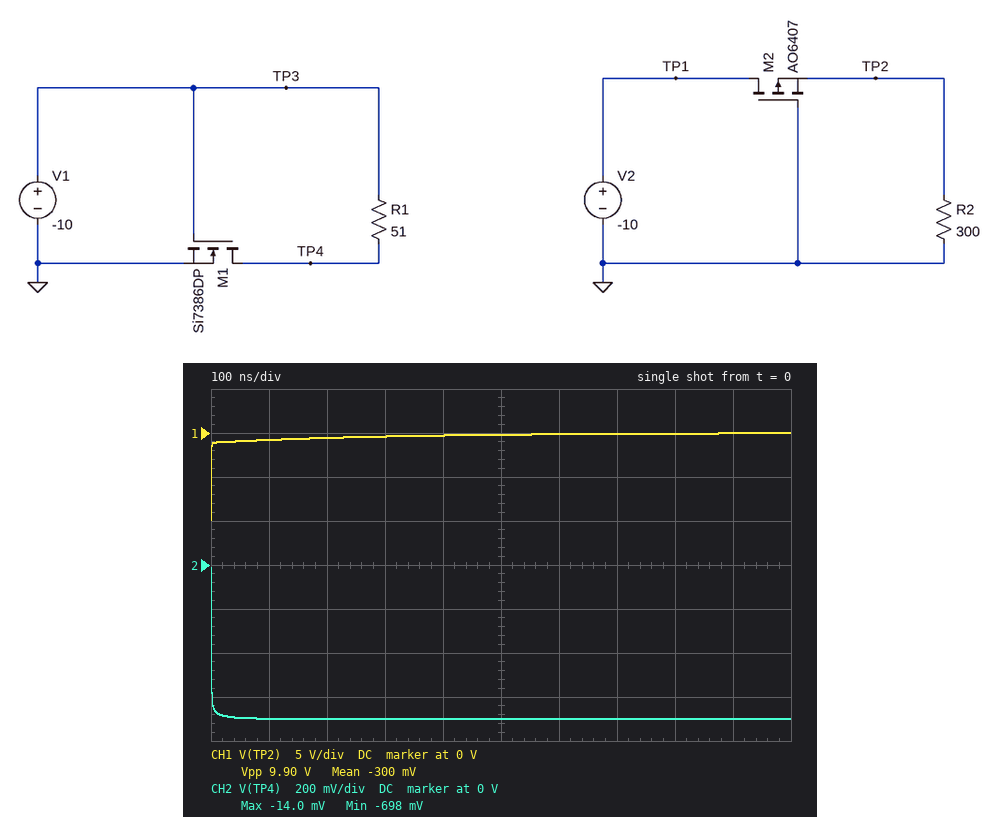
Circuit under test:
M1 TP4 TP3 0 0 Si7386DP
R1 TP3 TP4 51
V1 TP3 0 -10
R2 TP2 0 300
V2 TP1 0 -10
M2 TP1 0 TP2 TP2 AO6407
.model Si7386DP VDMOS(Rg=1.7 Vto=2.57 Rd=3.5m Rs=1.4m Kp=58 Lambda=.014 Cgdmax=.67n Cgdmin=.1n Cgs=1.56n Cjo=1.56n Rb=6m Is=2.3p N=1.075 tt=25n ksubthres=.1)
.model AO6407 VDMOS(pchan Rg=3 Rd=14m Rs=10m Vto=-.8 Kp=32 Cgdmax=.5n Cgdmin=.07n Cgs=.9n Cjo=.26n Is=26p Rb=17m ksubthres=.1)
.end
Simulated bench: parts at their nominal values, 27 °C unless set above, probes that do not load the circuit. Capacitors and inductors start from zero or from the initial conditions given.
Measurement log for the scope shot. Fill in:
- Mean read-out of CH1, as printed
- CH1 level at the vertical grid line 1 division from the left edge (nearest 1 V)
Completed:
-300 mV
-1 V
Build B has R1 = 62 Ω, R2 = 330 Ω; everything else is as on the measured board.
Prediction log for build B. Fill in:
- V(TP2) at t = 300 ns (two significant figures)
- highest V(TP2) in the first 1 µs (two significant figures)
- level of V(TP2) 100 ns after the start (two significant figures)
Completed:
-440 mV
-51 mV
-820 mV
